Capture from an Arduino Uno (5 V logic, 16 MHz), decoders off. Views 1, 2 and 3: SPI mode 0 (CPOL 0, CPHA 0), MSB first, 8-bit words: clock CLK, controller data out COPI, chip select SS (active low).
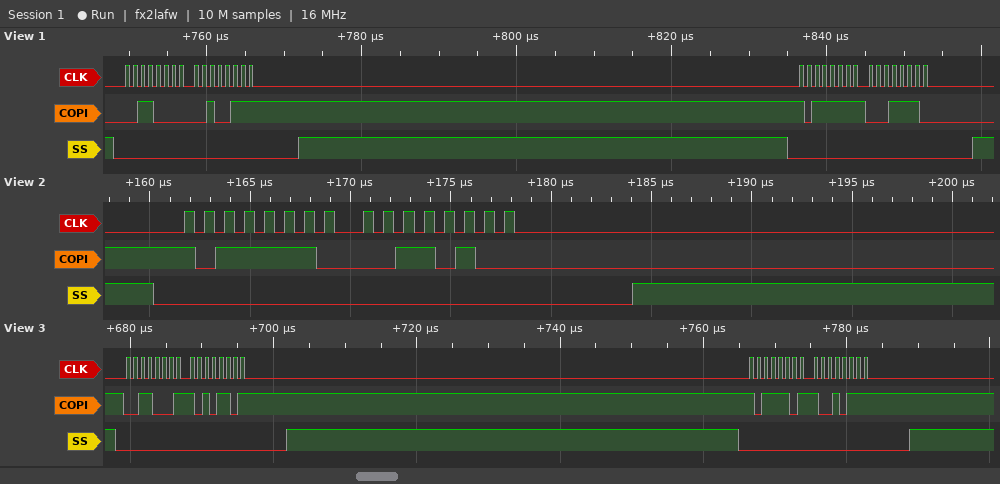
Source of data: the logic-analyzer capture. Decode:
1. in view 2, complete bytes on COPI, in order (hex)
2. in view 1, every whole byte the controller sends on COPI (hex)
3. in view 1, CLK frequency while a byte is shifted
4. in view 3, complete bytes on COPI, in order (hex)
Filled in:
BE 34
30 27 BF 1E
1 MHz
31 AD BD 97
